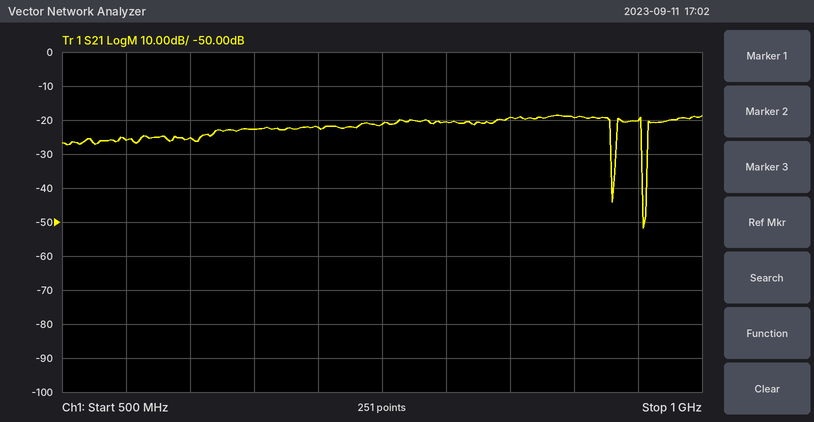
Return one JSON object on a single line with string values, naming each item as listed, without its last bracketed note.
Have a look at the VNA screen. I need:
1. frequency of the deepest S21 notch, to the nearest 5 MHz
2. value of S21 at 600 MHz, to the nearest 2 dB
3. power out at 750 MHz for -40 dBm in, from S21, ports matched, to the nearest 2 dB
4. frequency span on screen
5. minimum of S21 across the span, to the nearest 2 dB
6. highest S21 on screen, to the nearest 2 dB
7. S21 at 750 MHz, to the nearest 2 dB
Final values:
{"frequency of the deepest S21 notch, to the nearest 5 MHz": "955 MHz", "value of S21 at 600 MHz, to the nearest 2 dB": "-26 dB", "power out at 750 MHz for -40 dBm in, from S21, ports matched, to the nearest 2 dB": "-62 dBm", "frequency span on screen": "500 MHz", "minimum of S21 across the span, to the nearest 2 dB": "-52 dB", "highest S21 on screen, to the nearest 2 dB": "-18 dB", "S21 at 750 MHz, to the nearest 2 dB": "-22 dB"}
